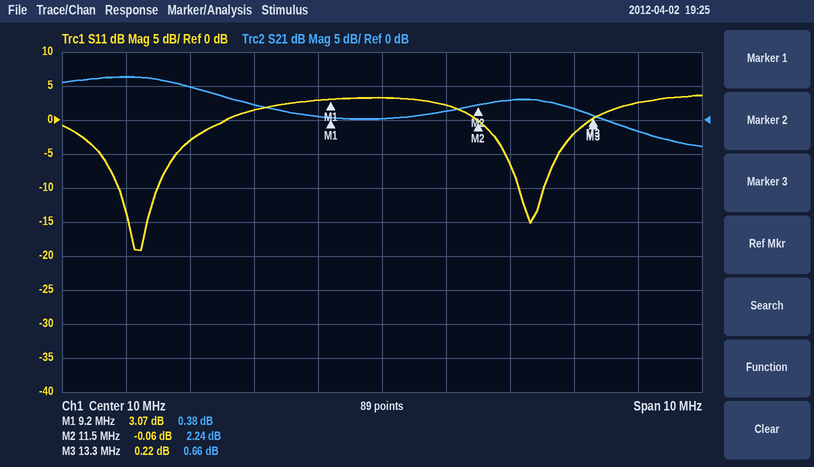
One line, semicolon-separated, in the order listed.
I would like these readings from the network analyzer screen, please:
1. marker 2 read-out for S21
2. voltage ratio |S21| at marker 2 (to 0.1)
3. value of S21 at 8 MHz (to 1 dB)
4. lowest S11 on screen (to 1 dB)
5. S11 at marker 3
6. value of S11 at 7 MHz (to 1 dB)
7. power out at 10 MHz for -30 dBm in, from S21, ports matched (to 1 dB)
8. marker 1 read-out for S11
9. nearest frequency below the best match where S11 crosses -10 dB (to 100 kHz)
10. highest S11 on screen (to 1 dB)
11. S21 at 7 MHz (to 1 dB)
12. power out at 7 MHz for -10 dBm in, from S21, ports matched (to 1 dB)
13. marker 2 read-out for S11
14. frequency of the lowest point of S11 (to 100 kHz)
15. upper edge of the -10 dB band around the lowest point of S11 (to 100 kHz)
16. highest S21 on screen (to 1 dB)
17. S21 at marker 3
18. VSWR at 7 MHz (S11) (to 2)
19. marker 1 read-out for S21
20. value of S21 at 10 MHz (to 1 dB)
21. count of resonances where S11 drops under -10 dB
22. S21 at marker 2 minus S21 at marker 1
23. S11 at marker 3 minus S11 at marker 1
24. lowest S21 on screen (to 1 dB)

2.24 dB; 1.3; 2 dB; -19 dB; 0.22 dB; -3 dB; -30 dBm; 3.07 dB; 5.9 MHz; 4 dB; 5 dB; -5 dBm; -0.06 dB; 6.2 MHz; 6.5 MHz; 6 dB; 0.66 dB; 6; 0.38 dB; 0 dB; 2; 1.86 dB; -2.85 dB; -4 dB
